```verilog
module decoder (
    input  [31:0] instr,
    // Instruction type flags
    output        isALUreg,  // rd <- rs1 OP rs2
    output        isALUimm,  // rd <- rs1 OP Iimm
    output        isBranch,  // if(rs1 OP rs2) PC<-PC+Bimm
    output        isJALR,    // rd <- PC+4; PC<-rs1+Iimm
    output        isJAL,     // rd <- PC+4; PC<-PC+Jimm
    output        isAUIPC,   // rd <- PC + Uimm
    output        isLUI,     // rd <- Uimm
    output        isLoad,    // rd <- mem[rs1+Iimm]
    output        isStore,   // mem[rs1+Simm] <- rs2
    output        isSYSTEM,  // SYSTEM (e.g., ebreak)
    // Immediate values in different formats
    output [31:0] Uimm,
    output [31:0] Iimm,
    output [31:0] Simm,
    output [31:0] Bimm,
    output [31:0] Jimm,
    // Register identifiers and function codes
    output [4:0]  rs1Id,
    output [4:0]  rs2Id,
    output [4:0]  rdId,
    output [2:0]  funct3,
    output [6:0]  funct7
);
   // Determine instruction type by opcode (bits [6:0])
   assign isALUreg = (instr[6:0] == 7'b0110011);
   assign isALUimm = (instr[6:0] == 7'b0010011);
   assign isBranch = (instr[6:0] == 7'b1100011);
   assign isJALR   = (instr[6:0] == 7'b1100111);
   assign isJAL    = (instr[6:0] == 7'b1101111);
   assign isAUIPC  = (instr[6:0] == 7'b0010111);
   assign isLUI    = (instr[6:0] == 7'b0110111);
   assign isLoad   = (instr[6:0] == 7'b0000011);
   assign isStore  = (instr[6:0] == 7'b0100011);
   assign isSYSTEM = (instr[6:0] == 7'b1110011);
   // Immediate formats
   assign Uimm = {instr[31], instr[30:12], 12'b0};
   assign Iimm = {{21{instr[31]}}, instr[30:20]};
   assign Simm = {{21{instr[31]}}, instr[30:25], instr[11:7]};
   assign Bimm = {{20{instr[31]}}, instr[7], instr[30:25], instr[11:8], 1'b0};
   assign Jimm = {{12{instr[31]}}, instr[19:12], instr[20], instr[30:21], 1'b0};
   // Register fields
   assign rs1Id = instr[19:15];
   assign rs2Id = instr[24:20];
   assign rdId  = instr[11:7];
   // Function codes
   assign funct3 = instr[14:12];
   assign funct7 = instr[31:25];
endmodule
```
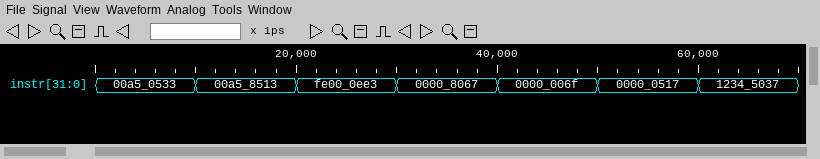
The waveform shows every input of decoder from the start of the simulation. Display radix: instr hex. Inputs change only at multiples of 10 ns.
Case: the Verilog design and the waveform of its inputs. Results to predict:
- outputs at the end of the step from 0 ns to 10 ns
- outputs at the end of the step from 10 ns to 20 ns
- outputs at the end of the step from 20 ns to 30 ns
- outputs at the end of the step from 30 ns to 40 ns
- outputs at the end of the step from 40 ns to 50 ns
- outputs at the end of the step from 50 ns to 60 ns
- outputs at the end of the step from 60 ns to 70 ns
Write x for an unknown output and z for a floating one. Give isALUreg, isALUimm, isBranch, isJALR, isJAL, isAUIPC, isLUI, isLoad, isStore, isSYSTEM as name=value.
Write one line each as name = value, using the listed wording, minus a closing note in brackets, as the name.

outputs at the end of the step from 0 ns to 10 ns = isALUreg=1, isALUimm=0, isBranch=0, isJALR=0, isJAL=0, isAUIPC=0, isLUI=0, isLoad=0, isStore=0, isSYSTEM=0
outputs at the end of the step from 10 ns to 20 ns = isALUreg=0, isALUimm=1, isBranch=0, isJALR=0, isJAL=0, isAUIPC=0, isLUI=0, isLoad=0, isStore=0, isSYSTEM=0
outputs at the end of the step from 20 ns to 30 ns = isALUreg=0, isALUimm=0, isBranch=1, isJALR=0, isJAL=0, isAUIPC=0, isLUI=0, isLoad=0, isStore=0, isSYSTEM=0
outputs at the end of the step from 30 ns to 40 ns = isALUreg=0, isALUimm=0, isBranch=0, isJALR=1, isJAL=0, isAUIPC=0, isLUI=0, isLoad=0, isStore=0, isSYSTEM=0
outputs at the end of the step from 40 ns to 50 ns = isALUreg=0, isALUimm=0, isBranch=0, isJALR=0, isJAL=1, isAUIPC=0, isLUI=0, isLoad=0, isStore=0, isSYSTEM=0
outputs at the end of the step from 50 ns to 60 ns = isALUreg=0, isALUimm=0, isBranch=0, isJALR=0, isJAL=0, isAUIPC=1, isLUI=0, isLoad=0, isStore=0, isSYSTEM=0
outputs at the end of the step from 60 ns to 70 ns = isALUreg=0, isALUimm=0, isBranch=0, isJALR=0, isJAL=0, isAUIPC=0, isLUI=1, isLoad=0, isStore=0, isSYSTEM=0
